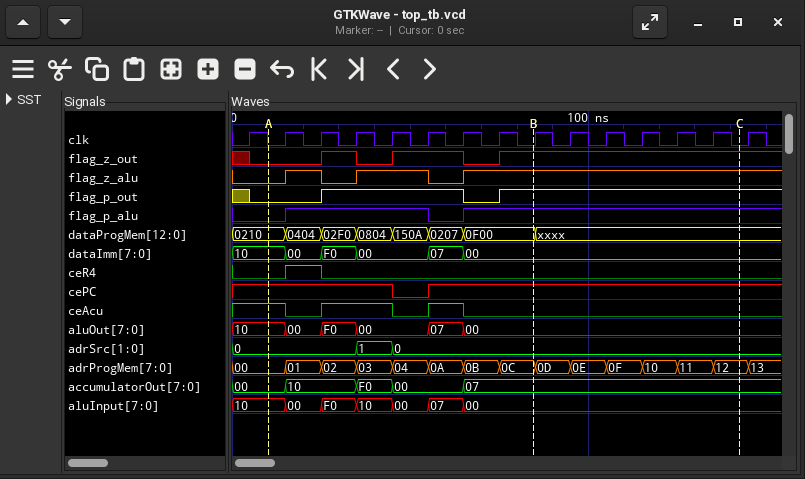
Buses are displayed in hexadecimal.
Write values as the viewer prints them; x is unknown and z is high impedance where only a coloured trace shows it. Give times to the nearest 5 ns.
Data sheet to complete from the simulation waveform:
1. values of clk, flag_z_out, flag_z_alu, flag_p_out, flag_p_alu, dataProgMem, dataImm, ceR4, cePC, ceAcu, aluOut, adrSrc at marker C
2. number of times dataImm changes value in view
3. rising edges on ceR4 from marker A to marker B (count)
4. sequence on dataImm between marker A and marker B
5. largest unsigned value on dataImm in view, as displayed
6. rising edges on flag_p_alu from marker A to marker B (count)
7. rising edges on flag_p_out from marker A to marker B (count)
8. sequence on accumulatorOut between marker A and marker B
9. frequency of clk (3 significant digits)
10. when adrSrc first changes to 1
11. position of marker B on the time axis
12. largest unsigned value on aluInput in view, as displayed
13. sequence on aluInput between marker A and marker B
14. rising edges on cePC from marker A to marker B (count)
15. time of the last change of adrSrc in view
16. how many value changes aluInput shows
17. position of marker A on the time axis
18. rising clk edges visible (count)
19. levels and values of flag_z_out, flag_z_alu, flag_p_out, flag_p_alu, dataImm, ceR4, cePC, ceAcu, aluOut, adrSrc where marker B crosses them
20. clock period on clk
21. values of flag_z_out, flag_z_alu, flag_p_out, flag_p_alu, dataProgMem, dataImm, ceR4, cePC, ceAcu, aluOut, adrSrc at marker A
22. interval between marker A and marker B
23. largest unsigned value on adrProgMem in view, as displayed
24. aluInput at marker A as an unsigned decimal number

clk=0, flag_z_out=1, flag_z_alu=1, flag_p_out=1, flag_p_alu=1, dataProgMem=xxxx, dataImm=00, ceR4=0, cePC=1, ceAcu=0, aluOut=00, adrSrc=0
5
1
10, 00, F0, 00, 07, 00
F0
2
2
00, 10, F0, 00, 07
100 MHz
35 ns
85 ns
F0
10, 00, F0, 10, 00, 07, 00
1
45 ns
6
10 ns
15
flag_z_out=1, flag_z_alu=1, flag_p_out=1, flag_p_alu=1, dataImm=00, ceR4=0, cePC=1, ceAcu=0, aluOut=00, adrSrc=0
10 ns
flag_z_out=0, flag_z_alu=0, flag_p_out=0, flag_p_alu=0, dataProgMem=0210, dataImm=10, ceR4=0, cePC=1, ceAcu=1, aluOut=10, adrSrc=0
75 ns
13
16
